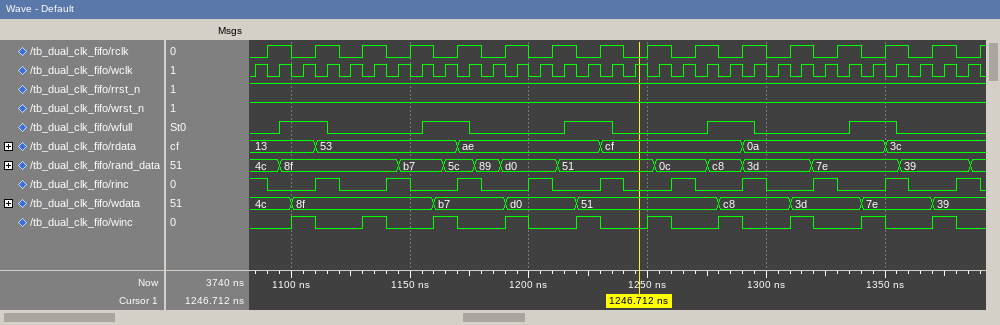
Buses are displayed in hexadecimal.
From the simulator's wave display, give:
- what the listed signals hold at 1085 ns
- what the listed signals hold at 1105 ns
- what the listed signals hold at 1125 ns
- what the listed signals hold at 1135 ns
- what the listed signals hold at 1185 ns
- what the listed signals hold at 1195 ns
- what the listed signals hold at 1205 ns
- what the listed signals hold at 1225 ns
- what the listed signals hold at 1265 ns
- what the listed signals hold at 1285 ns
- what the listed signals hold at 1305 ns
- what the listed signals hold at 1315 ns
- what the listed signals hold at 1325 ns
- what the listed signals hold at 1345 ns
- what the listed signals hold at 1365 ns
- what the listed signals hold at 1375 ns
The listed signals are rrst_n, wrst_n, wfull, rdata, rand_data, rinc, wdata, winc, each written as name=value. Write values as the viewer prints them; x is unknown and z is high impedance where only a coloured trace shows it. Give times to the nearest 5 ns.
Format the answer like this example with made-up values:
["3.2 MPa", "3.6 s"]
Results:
["rrst_n=1, wrst_n=1, wfull=0, rdata=13, rand_data=4c, rinc=1, wdata=4c, winc=0", "rrst_n=1, wrst_n=1, wfull=1, rdata=13, rand_data=8f, rinc=0, wdata=8f, winc=1", "rrst_n=1, wrst_n=1, wfull=0, rdata=53, rand_data=8f, rinc=0, wdata=8f, winc=0", "rrst_n=1, wrst_n=1, wfull=0, rdata=53, rand_data=8f, rinc=0, wdata=8f, winc=1", "rrst_n=1, wrst_n=1, wfull=0, rdata=ae, rand_data=89, rinc=0, wdata=b7, winc=0", "rrst_n=1, wrst_n=1, wfull=0, rdata=ae, rand_data=d0, rinc=0, wdata=d0, winc=1", "rrst_n=1, wrst_n=1, wfull=0, rdata=ae, rand_data=d0, rinc=1, wdata=d0, winc=0", "rrst_n=1, wrst_n=1, wfull=1, rdata=ae, rand_data=51, rinc=0, wdata=51, winc=1", "rrst_n=1, wrst_n=1, wfull=0, rdata=cf, rand_data=0c, rinc=1, wdata=51, winc=0", "rrst_n=1, wrst_n=1, wfull=1, rdata=cf, rand_data=c8, rinc=0, wdata=c8, winc=1", "rrst_n=1, wrst_n=1, wfull=0, rdata=0a, rand_data=3d, rinc=0, wdata=c8, winc=0", "rrst_n=1, wrst_n=1, wfull=0, rdata=0a, rand_data=3d, rinc=0, wdata=3d, winc=1", "rrst_n=1, wrst_n=1, wfull=0, rdata=0a, rand_data=7e, rinc=1, wdata=3d, winc=0", "rrst_n=1, wrst_n=1, wfull=1, rdata=0a, rand_data=7e, rinc=0, wdata=7e, winc=1", "rrst_n=1, wrst_n=1, wfull=0, rdata=3c, rand_data=39, rinc=0, wdata=7e, winc=0", "rrst_n=1, wrst_n=1, wfull=0, rdata=3c, rand_data=39, rinc=0, wdata=39, winc=1"]
